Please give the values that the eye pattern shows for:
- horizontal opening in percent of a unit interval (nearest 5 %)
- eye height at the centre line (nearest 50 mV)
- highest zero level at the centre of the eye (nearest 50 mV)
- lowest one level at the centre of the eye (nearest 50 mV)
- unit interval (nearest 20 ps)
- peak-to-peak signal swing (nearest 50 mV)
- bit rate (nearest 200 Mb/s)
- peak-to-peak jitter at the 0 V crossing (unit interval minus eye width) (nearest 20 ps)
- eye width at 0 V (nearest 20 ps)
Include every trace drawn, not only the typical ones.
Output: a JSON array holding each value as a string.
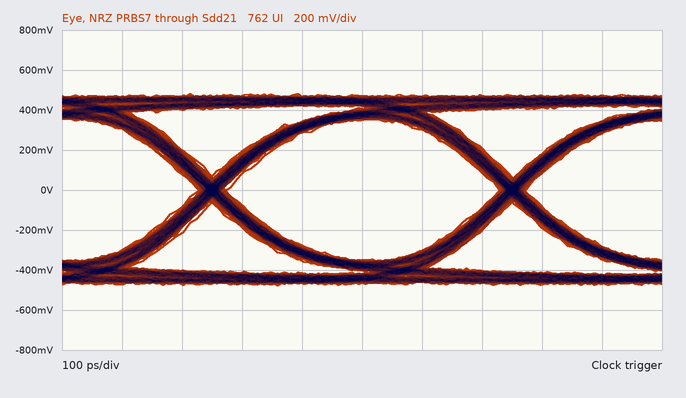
["90 %", "700 mV", "-350 mV", "350 mV", "500 ps", "950 mV", "2.0 Gb/s", "40 ps", "460 ps"]
